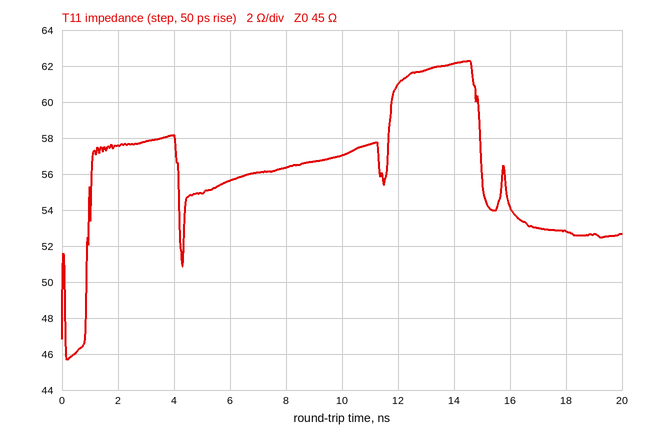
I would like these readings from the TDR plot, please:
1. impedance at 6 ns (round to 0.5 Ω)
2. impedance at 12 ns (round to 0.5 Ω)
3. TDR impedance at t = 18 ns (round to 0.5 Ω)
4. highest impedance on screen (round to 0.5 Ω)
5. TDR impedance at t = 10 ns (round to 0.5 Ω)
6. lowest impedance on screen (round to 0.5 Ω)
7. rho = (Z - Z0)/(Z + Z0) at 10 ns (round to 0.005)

55.5 Ω
61.0 Ω
53.0 Ω
62.5 Ω
57.0 Ω
45.5 Ω
+0.120
